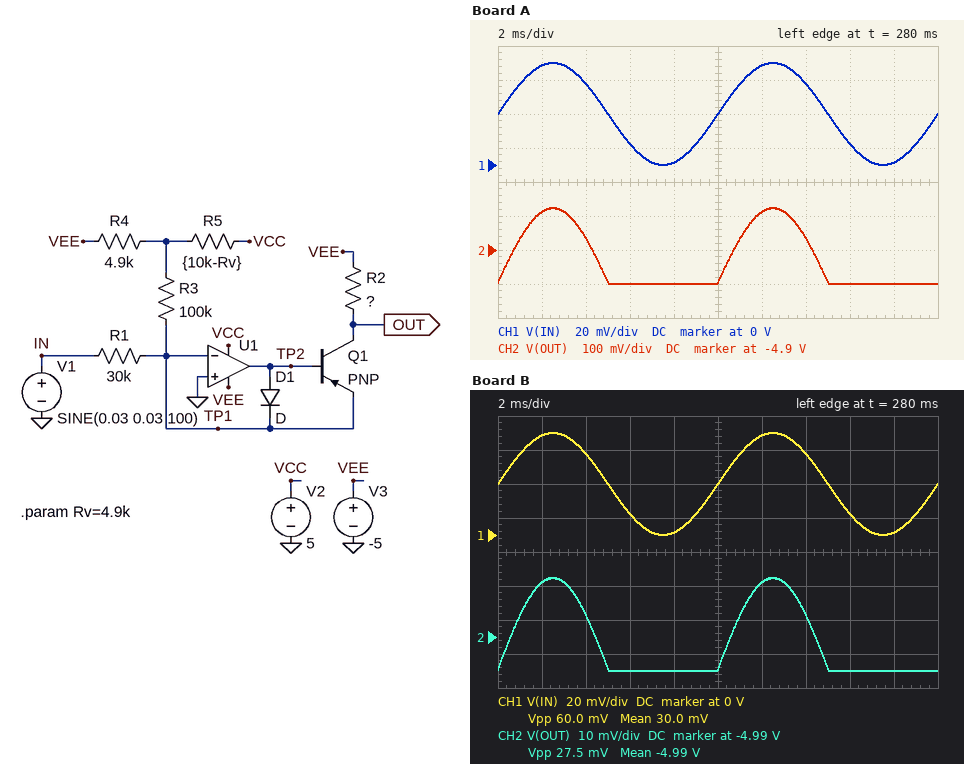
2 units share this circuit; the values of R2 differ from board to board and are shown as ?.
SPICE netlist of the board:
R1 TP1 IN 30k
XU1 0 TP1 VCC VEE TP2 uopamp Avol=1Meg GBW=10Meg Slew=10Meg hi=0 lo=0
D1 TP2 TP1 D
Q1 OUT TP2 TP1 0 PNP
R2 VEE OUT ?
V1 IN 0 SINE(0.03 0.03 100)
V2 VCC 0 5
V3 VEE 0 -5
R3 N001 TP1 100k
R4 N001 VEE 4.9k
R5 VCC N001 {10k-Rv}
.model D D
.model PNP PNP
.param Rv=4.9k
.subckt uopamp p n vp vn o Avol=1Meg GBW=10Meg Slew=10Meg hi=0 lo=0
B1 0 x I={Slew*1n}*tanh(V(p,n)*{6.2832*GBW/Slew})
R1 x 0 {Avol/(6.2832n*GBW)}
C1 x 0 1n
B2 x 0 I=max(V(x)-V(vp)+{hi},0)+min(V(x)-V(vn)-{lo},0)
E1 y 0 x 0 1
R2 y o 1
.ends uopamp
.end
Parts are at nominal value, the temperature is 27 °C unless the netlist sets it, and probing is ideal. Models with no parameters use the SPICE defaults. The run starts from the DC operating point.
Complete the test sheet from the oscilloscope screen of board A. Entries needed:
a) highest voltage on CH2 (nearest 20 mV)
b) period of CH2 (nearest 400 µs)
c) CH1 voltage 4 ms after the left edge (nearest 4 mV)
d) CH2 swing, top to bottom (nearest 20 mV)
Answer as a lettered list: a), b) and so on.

a) -4.78 V
b) 10.0 ms
c) 48 mV
d) 220 mV
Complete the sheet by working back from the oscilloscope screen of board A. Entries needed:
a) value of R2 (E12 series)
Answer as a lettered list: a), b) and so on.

a) 220 kΩ
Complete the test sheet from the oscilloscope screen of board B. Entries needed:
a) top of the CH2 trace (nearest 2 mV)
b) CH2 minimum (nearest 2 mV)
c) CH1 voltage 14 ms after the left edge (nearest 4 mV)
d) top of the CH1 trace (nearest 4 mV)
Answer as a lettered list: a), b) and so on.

a) -4.972 V
b) -5.000 V
c) 48 mV
d) 60 mV
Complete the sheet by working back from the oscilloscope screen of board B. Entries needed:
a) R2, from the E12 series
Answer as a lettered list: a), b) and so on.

a) 27 kΩ
